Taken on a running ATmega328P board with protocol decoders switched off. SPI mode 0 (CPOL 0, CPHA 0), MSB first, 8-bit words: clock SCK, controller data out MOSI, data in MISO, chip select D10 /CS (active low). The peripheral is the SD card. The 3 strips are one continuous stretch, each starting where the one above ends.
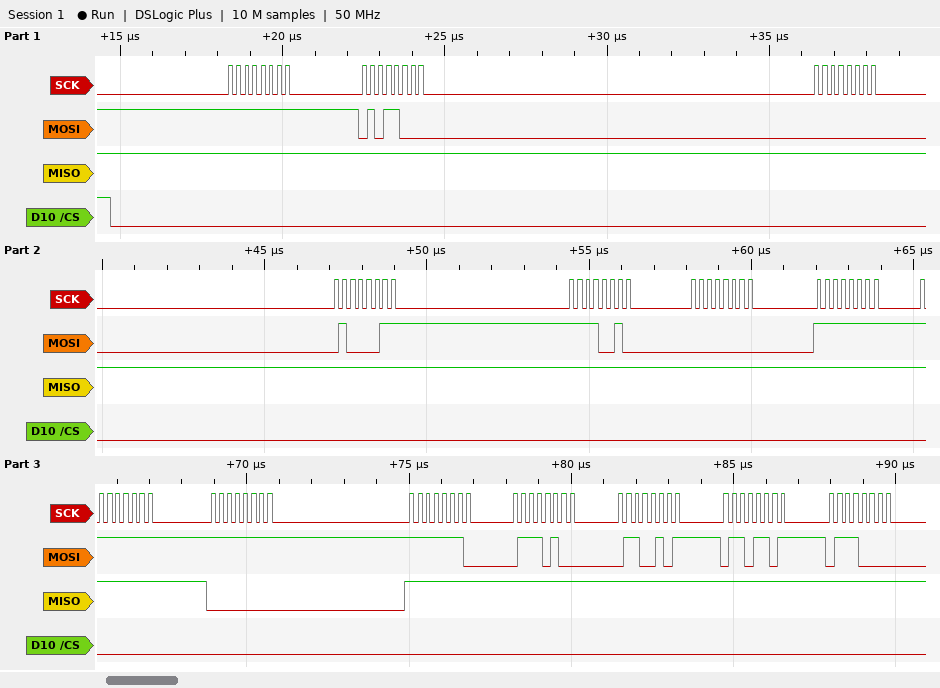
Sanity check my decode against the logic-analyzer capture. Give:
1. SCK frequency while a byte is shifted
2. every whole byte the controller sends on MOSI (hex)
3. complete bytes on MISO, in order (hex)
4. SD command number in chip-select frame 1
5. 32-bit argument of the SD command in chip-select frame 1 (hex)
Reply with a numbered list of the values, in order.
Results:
1. 4 MHz
2. 0xFF 0x58 0x00 0x43 0xF2 0x00 0xFF 0xFF 0xFF 0xFE 0x74 0x65 0x6D 0x70
3. 0xFF 0xFF 0xFF 0xFF 0xFF 0xFF 0xFF 0xFF 0x00 0xFF 0xFF 0xFF 0xFF 0xFF
4. CMD24
5. 0x0043F200
